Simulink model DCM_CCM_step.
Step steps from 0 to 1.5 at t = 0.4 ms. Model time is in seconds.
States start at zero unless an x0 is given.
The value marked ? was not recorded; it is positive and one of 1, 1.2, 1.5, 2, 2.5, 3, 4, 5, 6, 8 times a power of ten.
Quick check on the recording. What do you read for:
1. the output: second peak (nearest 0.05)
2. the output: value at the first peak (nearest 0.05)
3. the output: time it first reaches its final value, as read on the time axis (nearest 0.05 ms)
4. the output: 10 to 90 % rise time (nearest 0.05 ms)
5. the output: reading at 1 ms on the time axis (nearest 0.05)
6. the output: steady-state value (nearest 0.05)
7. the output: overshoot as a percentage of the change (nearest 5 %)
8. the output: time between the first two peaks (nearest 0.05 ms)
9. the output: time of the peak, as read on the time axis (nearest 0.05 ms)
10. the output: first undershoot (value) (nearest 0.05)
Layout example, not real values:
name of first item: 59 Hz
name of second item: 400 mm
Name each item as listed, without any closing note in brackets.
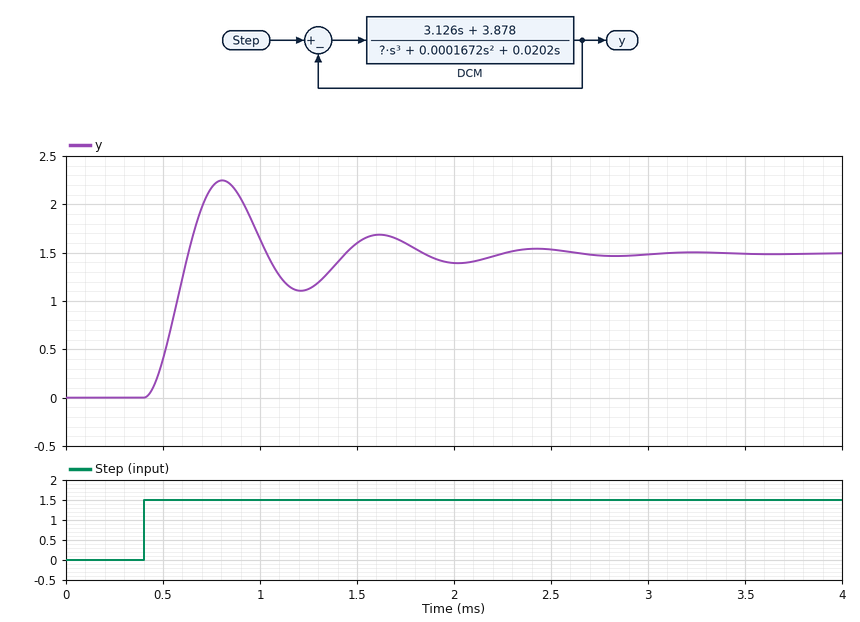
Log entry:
the output: second peak: 1.70
the output: value at the first peak: 2.25
the output: time it first reaches its final value, as read on the time axis: 0.65 ms
the output: 10 to 90 % rise time: 0.15 ms
the output: reading at 1 ms on the time axis: 1.65
the output: steady-state value: 1.50
the output: overshoot as a percentage of the change: 50 %
the output: time between the first two peaks: 0.80 ms
the output: time of the peak, as read on the time axis: 0.80 ms
the output: first undershoot (value): 1.10
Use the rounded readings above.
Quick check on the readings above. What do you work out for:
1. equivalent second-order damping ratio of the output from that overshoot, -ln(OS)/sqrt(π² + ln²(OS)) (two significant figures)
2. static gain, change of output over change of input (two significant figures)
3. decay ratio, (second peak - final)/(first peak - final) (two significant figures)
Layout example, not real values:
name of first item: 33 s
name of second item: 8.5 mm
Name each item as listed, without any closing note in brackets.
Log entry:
equivalent second-order damping ratio of the output from that overshoot, -ln(OS)/sqrt(π² + ln²(OS)): 0.22
static gain, change of output over change of input: 1.0
decay ratio, (second peak - final)/(first peak - final): 0.27
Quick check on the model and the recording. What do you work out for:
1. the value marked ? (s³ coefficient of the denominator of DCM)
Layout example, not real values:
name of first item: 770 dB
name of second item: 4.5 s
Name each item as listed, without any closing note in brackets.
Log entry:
the value marked ?: 5e-08
